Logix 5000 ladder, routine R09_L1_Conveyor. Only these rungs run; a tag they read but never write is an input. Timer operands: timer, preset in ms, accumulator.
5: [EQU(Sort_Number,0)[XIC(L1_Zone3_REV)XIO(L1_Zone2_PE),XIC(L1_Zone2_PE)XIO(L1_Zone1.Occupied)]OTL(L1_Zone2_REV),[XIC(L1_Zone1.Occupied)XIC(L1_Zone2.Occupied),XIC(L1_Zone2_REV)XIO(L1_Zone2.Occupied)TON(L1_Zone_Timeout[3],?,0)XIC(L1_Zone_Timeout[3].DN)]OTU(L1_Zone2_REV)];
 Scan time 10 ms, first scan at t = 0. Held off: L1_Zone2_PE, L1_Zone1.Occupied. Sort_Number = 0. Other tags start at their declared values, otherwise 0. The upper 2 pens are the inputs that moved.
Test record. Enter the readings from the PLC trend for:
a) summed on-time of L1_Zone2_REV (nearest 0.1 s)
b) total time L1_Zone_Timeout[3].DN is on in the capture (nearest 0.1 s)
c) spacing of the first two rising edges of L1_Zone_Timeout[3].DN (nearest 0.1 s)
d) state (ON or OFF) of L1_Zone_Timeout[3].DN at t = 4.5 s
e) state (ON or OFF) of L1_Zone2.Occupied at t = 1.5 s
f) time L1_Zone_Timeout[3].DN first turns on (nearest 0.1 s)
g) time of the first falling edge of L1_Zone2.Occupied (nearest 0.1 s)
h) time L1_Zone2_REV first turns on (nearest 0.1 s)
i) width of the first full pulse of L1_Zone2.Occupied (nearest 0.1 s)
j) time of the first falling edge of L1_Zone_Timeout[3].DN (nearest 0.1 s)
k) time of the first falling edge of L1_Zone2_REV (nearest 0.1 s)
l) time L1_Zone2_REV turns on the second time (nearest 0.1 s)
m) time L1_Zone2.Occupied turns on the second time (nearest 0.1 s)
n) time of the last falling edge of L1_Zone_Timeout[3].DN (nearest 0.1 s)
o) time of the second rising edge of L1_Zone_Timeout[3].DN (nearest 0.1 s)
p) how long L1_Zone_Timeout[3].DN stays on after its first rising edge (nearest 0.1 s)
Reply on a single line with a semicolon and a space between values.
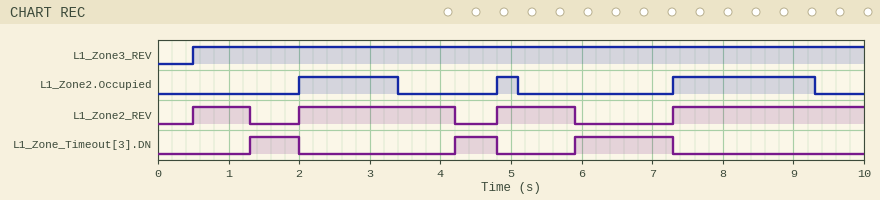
6.8 s; 2.7 s; 2.9 s; ON; OFF; 1.3 s; 3.4 s; 0.5 s; 1.4 s; 2.0 s; 1.3 s; 2.0 s; 4.8 s; 7.3 s; 4.2 s; 0.7 s
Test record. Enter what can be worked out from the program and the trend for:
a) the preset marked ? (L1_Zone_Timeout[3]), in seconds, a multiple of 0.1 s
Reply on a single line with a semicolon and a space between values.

0.8 s
